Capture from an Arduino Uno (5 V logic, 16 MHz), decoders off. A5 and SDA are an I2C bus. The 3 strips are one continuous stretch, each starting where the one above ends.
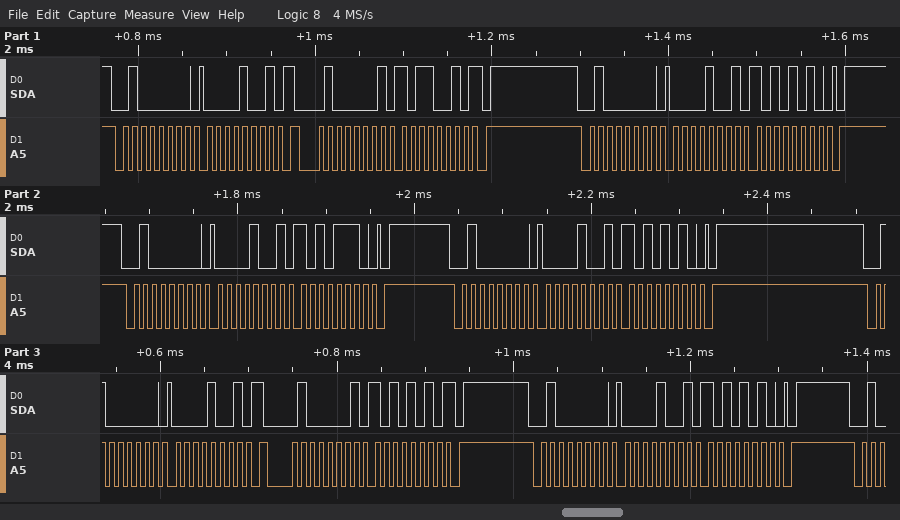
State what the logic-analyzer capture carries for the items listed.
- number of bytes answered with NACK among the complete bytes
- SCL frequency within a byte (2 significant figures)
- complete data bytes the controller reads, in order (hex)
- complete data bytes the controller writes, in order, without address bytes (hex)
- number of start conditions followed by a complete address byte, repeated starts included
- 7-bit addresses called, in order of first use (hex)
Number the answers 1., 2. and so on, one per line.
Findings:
1. 2
2. 100 kHz
3. B2 AA
4. 09 09 AA 09 AE 09 AA 09 09 AA
5. 8
6. 0x20
